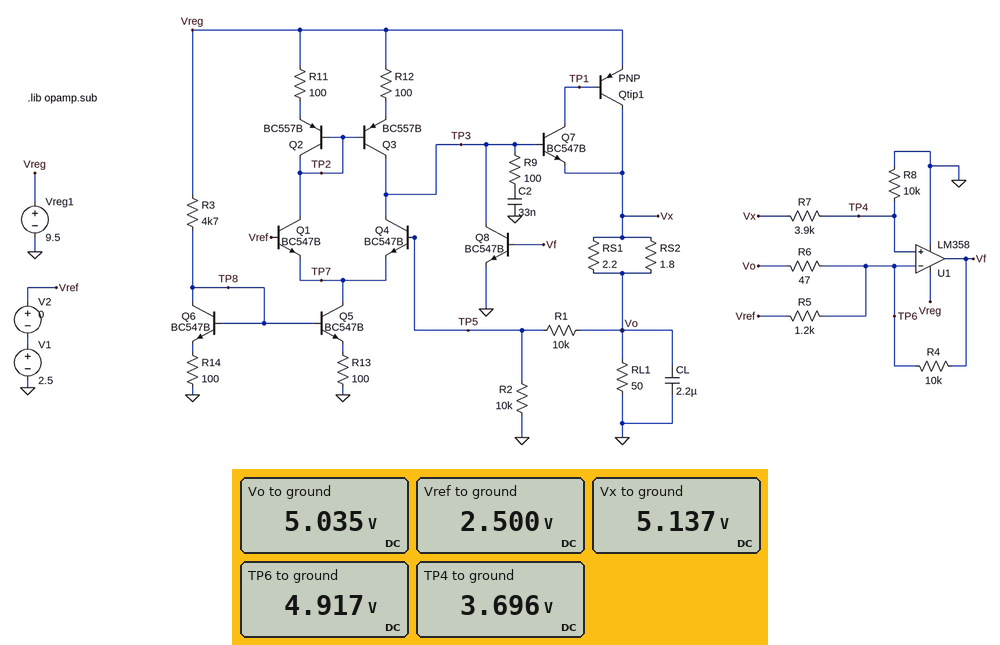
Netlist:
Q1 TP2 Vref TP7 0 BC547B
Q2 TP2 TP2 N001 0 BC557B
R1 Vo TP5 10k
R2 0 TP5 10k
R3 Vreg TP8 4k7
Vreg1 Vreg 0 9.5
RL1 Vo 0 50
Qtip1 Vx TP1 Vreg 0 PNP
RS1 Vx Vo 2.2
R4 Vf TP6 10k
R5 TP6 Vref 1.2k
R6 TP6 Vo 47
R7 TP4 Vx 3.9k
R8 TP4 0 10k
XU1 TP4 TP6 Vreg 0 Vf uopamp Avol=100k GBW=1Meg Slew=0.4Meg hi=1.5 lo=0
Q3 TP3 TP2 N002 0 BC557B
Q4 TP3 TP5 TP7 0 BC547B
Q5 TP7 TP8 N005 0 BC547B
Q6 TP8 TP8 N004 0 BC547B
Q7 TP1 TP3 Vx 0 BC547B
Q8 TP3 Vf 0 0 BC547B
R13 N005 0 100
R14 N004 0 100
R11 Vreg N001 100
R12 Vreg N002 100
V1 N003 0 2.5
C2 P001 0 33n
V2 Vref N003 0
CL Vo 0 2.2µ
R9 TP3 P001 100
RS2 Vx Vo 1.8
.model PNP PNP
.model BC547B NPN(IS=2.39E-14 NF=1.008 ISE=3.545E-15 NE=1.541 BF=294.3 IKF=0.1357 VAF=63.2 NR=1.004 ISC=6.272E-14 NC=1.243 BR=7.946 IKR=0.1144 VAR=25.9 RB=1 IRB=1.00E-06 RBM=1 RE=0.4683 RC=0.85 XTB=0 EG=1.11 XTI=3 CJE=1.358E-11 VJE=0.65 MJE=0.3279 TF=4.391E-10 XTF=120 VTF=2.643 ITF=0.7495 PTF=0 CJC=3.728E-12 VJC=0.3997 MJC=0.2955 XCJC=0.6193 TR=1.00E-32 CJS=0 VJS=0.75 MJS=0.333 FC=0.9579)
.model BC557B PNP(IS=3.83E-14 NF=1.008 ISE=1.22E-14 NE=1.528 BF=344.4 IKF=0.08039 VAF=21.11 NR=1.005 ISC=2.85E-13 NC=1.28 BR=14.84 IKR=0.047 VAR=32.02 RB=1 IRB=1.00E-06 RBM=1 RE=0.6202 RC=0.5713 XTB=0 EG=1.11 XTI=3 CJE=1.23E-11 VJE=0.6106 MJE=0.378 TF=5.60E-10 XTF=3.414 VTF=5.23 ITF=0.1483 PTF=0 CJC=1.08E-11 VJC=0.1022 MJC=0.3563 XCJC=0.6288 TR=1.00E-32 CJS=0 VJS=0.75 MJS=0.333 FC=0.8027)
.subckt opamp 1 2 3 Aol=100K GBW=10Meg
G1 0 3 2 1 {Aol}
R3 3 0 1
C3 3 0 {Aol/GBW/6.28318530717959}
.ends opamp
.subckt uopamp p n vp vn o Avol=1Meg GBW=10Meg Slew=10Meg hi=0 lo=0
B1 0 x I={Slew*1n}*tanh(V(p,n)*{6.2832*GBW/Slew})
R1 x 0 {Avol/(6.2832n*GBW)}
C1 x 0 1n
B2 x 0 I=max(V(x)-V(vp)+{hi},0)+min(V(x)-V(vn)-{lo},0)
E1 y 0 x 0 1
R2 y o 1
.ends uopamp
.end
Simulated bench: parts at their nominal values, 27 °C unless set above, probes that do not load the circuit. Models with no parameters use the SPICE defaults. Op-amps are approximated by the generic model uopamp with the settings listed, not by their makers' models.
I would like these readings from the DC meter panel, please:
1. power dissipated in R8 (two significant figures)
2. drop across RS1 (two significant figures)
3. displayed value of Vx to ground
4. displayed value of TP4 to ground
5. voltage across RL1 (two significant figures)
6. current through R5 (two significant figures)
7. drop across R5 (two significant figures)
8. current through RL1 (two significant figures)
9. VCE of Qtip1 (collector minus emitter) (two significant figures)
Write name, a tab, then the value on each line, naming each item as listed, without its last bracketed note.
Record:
power dissipated in R8	1.4 mW
drop across RS1	100 mV
displayed value of Vx to ground	5.137 V
displayed value of TP4 to ground	3.696 V
voltage across RL1	5.0 V
current through R5	2.0 mA
drop across R5	2.4 V
current through RL1	100 mA
VCE of Qtip1 (collector minus emitter)	-4.4 V
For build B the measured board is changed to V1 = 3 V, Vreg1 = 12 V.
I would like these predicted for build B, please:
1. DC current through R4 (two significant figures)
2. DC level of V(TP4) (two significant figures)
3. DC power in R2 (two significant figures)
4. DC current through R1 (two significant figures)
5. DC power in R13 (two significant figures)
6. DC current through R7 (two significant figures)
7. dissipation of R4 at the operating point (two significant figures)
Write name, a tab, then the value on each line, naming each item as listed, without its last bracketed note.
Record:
DC current through R4	590 µA
DC level of V(TP4)	4.4 V
DC power in R2	900 µW
DC current through R1	300 µA
DC power in R13	560 µW
DC current through R7	440 µA
dissipation of R4 at the operating point	3.5 mW
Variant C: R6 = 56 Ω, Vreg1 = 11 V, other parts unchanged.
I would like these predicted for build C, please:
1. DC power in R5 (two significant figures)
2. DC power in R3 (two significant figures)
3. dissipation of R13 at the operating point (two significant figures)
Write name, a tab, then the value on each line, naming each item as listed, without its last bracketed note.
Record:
DC power in R5	4.8 mW
DC power in R3	22 mW
dissipation of R13 at the operating point	460 µW
